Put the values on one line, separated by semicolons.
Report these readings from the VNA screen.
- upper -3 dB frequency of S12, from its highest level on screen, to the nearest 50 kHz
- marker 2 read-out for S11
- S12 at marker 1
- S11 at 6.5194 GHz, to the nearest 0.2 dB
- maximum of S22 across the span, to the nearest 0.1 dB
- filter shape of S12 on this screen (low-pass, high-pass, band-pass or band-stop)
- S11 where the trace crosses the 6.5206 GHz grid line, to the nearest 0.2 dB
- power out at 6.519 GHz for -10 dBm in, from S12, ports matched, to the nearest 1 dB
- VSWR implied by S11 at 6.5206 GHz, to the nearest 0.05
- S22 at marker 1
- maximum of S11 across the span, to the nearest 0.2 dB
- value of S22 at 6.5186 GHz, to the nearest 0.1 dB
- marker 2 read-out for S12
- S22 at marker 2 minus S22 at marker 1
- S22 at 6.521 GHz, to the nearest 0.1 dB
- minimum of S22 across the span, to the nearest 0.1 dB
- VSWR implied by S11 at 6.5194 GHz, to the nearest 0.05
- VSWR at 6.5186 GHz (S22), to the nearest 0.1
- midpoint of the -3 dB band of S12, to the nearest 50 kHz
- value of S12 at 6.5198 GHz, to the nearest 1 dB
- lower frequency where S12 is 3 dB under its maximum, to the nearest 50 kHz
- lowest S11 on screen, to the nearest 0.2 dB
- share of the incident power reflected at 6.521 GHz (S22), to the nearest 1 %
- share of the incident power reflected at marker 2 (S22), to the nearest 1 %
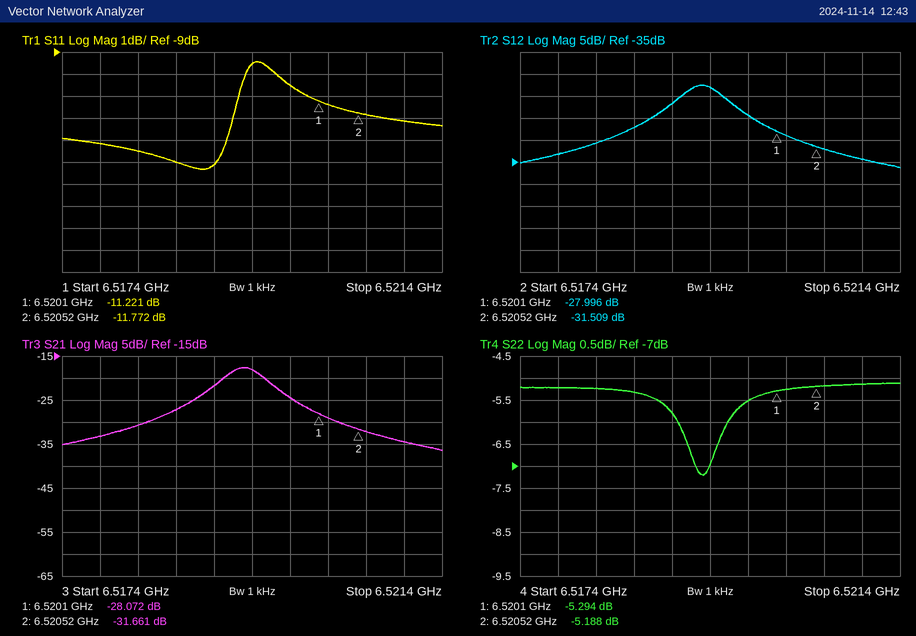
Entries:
6.51955 GHz; -11.772 dB; -27.996 dB; -9.6 dB; -5.1 dB; band-pass; -11.8 dB; -32 dBm; 1.70; -5.294 dB; -9.4 dB; -5.3 dB; -31.509 dB; 0.106 dB; -5.1 dB; -7.2 dB; 2.00; 3.4; 6.51930 GHz; -24 dB; 6.51905 GHz; -14.4 dB; 31 %; 30 %
